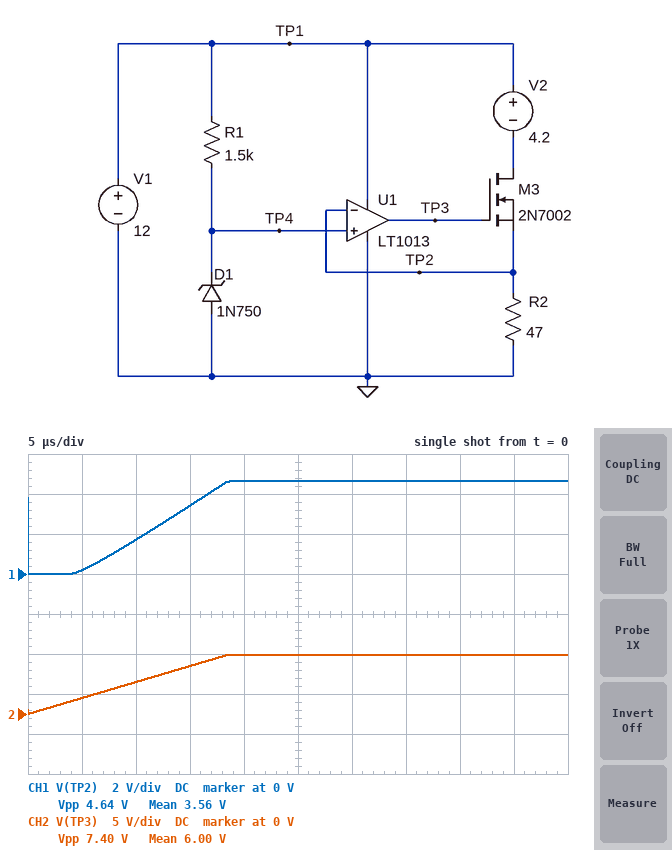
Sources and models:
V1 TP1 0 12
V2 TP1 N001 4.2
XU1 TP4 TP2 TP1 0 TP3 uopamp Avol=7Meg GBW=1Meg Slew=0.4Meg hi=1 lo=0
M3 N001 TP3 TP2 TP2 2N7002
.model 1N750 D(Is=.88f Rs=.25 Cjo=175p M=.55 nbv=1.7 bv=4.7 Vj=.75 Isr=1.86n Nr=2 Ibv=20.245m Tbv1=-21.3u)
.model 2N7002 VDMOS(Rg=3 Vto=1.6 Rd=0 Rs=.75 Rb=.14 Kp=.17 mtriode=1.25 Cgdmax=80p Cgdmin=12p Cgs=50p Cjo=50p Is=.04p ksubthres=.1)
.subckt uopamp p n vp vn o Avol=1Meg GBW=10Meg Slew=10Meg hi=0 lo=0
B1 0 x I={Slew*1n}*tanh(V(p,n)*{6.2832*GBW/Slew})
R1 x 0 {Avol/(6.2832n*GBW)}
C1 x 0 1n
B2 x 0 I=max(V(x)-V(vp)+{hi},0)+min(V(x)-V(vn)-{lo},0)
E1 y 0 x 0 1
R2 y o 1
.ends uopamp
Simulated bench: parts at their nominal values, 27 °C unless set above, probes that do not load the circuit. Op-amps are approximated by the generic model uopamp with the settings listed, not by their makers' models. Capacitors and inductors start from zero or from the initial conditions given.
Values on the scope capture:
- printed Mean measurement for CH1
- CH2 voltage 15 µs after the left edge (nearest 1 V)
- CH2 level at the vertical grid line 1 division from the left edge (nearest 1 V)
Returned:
3.56 V
6 V
2 V
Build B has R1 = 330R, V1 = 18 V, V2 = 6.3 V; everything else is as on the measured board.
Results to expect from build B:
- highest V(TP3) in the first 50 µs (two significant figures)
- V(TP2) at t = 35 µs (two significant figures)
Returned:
7.5 V
4.7 V
